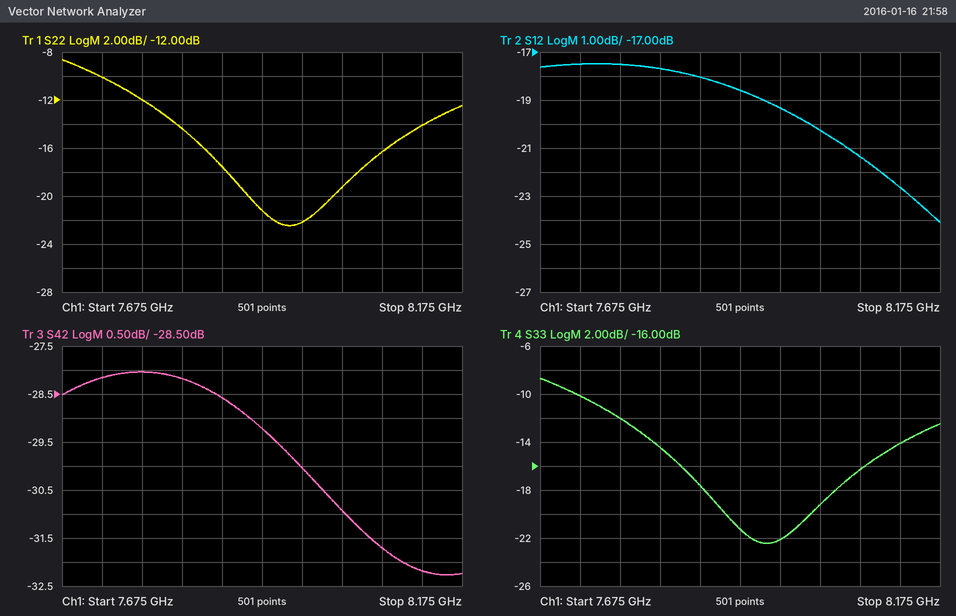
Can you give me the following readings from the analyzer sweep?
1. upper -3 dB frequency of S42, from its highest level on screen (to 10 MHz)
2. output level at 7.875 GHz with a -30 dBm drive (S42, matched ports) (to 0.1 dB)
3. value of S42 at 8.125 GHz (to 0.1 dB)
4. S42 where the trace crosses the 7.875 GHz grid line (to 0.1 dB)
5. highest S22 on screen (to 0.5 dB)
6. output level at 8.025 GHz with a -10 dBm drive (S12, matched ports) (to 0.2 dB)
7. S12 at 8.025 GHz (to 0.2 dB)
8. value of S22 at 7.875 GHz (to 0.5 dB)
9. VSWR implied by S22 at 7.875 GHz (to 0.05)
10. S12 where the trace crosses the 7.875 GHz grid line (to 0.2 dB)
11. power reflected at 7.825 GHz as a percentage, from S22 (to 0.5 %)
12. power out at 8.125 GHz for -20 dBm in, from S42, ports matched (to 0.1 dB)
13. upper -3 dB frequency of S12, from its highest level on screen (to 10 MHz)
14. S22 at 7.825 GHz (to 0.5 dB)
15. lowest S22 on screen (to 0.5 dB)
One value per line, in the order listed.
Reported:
8.03 GHz
-58.6 dBm
-32.2 dB
-28.6 dB
-8.5 dB
-30.2 dBm
-20.2 dB
-17.5 dB
1.30
-18.0 dB
3.5 %
-52.2 dBm
8.04 GHz
-14.5 dB
-22.5 dB
